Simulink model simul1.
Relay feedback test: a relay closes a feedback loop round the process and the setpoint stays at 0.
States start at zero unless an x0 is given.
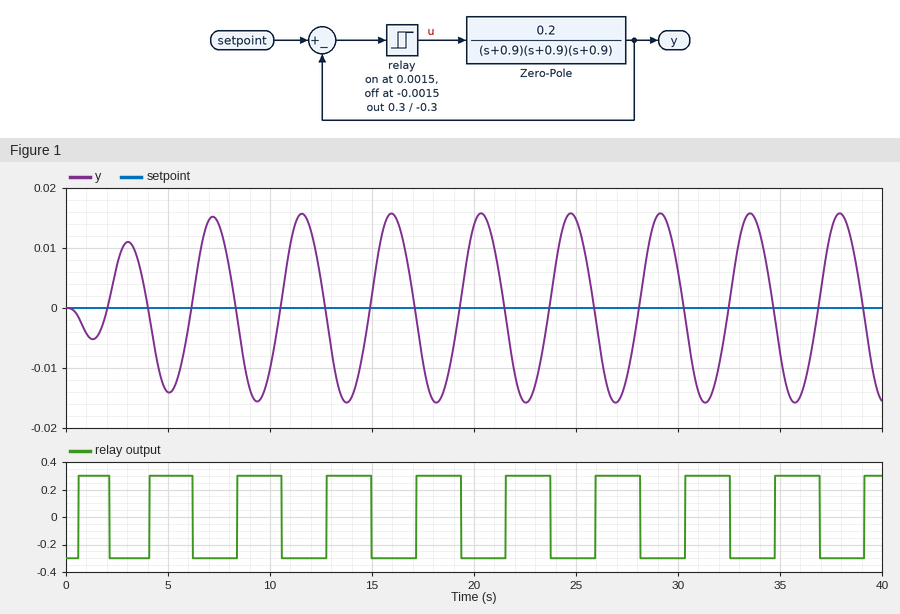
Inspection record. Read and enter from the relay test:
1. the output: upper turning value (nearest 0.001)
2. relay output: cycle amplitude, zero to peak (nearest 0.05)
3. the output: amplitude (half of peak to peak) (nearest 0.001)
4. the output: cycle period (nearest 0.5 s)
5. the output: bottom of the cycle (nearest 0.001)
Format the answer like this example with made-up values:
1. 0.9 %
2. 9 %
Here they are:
1. 0.016
2. 0.30
3. 0.016
4. 4.5 s
5. -0.016
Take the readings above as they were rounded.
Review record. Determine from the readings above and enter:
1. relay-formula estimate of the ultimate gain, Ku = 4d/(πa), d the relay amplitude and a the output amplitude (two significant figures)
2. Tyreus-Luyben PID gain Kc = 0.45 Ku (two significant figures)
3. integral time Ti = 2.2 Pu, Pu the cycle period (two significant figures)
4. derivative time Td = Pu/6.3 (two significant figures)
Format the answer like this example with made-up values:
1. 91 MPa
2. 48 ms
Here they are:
1. 24
2. 11
3. 9.9 s
4. 0.71 s
